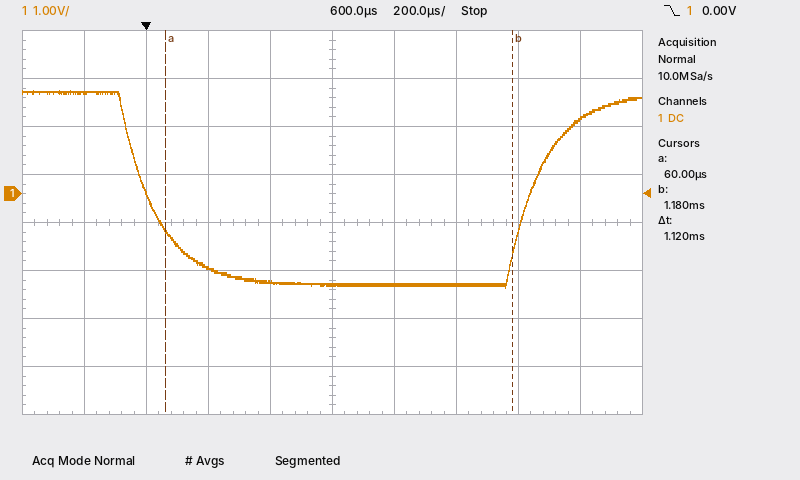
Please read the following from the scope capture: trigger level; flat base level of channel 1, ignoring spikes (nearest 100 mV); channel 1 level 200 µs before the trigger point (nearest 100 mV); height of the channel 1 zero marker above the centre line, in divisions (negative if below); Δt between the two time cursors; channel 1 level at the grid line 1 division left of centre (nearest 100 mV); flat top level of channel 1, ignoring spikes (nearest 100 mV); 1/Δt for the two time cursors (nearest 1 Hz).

0.00 V
-1.9 V
2.1 V
+0.6 div
1.12 ms
-1.8 V
2.1 V
893 Hz
